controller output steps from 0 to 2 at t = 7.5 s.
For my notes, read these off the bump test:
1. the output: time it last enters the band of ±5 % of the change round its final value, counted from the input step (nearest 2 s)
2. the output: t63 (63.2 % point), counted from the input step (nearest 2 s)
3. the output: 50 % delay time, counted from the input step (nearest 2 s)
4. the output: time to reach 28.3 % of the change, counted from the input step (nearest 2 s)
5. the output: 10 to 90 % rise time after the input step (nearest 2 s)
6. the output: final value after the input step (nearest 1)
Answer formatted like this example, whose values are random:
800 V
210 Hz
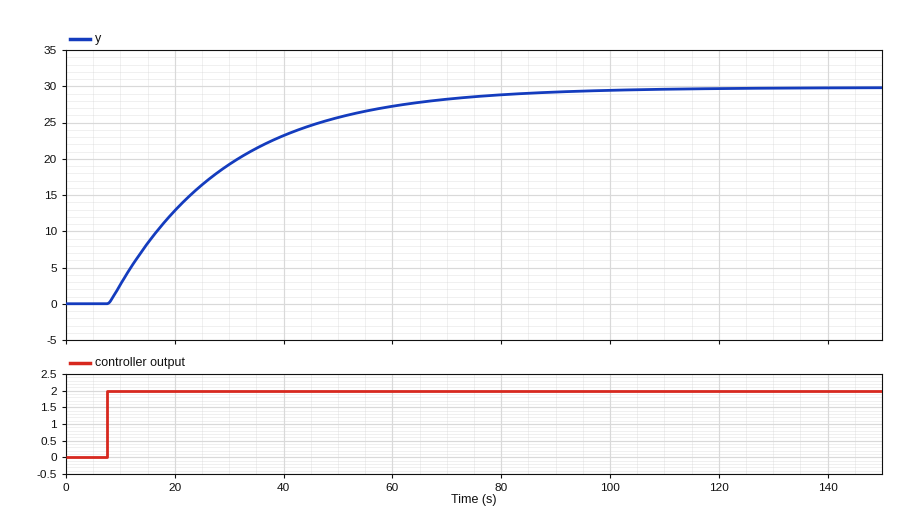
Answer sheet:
64 s
22 s
16 s
8 s
46 s
30
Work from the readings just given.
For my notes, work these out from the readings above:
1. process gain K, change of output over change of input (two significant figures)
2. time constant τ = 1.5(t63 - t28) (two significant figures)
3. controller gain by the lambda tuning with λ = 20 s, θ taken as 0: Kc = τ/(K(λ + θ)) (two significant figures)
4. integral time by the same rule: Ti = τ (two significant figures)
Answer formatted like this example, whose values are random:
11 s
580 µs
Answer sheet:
15
21 s
0.070
21 s
